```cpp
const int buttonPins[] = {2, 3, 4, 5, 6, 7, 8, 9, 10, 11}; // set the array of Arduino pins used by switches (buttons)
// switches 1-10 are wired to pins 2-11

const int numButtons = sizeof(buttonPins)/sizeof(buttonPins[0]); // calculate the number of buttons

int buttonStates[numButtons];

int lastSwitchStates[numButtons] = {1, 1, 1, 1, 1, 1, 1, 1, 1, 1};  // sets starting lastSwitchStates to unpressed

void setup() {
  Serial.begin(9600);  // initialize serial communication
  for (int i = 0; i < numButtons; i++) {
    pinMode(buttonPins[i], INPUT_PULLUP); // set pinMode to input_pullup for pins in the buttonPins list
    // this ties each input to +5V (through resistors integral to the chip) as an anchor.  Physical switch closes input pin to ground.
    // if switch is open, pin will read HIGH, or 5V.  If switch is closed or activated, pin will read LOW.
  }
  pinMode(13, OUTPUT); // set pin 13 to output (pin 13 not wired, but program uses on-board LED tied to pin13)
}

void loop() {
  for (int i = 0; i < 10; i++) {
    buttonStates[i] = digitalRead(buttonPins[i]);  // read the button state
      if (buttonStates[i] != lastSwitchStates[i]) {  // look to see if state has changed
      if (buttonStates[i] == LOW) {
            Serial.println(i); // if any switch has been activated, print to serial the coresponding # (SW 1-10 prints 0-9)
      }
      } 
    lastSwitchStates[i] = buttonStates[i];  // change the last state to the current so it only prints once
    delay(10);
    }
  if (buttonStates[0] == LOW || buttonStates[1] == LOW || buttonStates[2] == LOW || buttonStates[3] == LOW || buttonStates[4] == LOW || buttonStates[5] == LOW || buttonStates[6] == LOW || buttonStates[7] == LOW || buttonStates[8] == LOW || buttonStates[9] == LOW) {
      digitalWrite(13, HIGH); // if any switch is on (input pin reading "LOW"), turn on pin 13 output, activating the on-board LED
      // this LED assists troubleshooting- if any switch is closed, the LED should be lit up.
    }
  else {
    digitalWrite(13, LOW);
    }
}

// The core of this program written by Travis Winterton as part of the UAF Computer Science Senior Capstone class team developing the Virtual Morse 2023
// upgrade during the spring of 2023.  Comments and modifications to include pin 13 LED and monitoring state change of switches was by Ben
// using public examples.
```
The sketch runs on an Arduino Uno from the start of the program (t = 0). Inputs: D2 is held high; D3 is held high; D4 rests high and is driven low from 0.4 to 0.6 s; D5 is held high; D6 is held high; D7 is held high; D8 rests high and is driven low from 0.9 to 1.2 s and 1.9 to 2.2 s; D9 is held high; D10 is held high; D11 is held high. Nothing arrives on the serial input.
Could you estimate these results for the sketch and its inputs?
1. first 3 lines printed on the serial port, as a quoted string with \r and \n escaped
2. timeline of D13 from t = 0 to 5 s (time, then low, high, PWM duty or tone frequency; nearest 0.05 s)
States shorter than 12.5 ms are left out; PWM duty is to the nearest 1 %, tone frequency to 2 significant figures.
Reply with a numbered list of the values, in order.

1. "2\r\n6\r\n6\r\n"
2. 0 s low; 0.5 s high; 0.7 s low; 1 s high; 1.3 s low; 2 s high; 2.3 s low
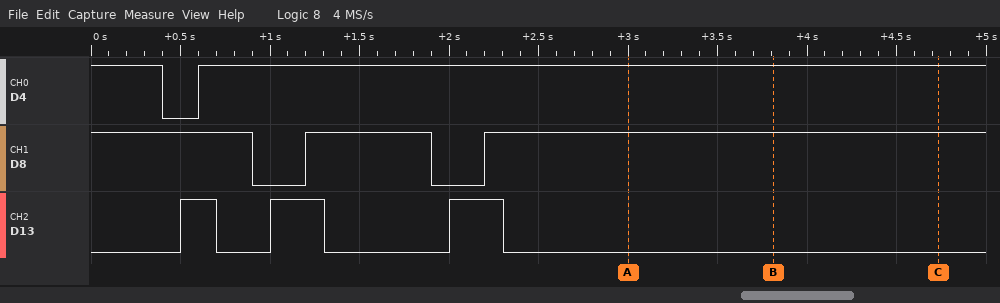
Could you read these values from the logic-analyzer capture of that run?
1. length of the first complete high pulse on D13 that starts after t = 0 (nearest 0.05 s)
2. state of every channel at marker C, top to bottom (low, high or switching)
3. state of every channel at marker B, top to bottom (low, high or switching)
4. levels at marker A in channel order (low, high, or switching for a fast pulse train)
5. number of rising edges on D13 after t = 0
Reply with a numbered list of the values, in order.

1. 0.20 s
2. D4 high, D8 high, D13 low
3. D4 high, D8 high, D13 low
4. D4 high, D8 high, D13 low
5. 3
